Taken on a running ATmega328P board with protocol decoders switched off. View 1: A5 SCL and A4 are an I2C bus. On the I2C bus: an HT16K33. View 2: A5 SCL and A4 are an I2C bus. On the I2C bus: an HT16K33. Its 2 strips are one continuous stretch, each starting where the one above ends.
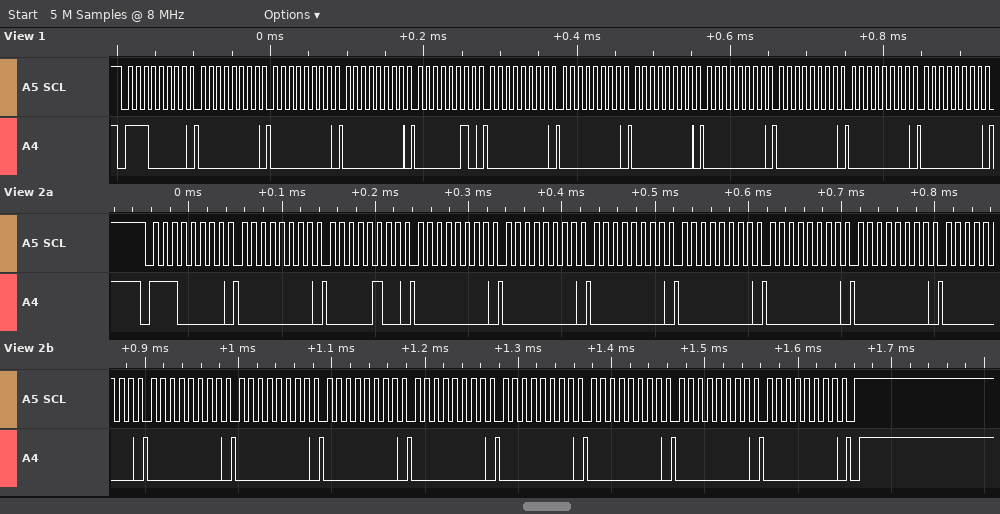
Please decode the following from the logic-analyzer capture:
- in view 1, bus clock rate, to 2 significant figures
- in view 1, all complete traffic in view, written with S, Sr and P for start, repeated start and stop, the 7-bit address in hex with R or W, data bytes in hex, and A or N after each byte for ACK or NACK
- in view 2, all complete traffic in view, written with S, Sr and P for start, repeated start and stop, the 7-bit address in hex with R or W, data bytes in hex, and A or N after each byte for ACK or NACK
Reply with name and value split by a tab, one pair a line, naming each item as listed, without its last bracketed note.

in view 1, bus clock rate, to 2 significant figures	100 kHz
in view 1, all complete traffic in view, written with S, Sr and P for start, repeated start and stop, the 7-bit address in hex with R or W, data bytes in hex, and A or N after each byte for ACK or NACK	S 70W A 00 A 00 A 00 A 02 A 00 A 00 A 00 A 00 A 00 A 00 A 00 A
in view 2, all complete traffic in view, written with S, Sr and P for start, repeated start and stop, the 7-bit address in hex with R or W, data bytes in hex, and A or N after each byte for ACK or NACK	S 70W A 00 A 04 A 00 A 00 A 00 A 00 A 00 A 00 A 00 A 00 A 00 A 00 A 00 A 00 A 00 A 00 A 00 A P
